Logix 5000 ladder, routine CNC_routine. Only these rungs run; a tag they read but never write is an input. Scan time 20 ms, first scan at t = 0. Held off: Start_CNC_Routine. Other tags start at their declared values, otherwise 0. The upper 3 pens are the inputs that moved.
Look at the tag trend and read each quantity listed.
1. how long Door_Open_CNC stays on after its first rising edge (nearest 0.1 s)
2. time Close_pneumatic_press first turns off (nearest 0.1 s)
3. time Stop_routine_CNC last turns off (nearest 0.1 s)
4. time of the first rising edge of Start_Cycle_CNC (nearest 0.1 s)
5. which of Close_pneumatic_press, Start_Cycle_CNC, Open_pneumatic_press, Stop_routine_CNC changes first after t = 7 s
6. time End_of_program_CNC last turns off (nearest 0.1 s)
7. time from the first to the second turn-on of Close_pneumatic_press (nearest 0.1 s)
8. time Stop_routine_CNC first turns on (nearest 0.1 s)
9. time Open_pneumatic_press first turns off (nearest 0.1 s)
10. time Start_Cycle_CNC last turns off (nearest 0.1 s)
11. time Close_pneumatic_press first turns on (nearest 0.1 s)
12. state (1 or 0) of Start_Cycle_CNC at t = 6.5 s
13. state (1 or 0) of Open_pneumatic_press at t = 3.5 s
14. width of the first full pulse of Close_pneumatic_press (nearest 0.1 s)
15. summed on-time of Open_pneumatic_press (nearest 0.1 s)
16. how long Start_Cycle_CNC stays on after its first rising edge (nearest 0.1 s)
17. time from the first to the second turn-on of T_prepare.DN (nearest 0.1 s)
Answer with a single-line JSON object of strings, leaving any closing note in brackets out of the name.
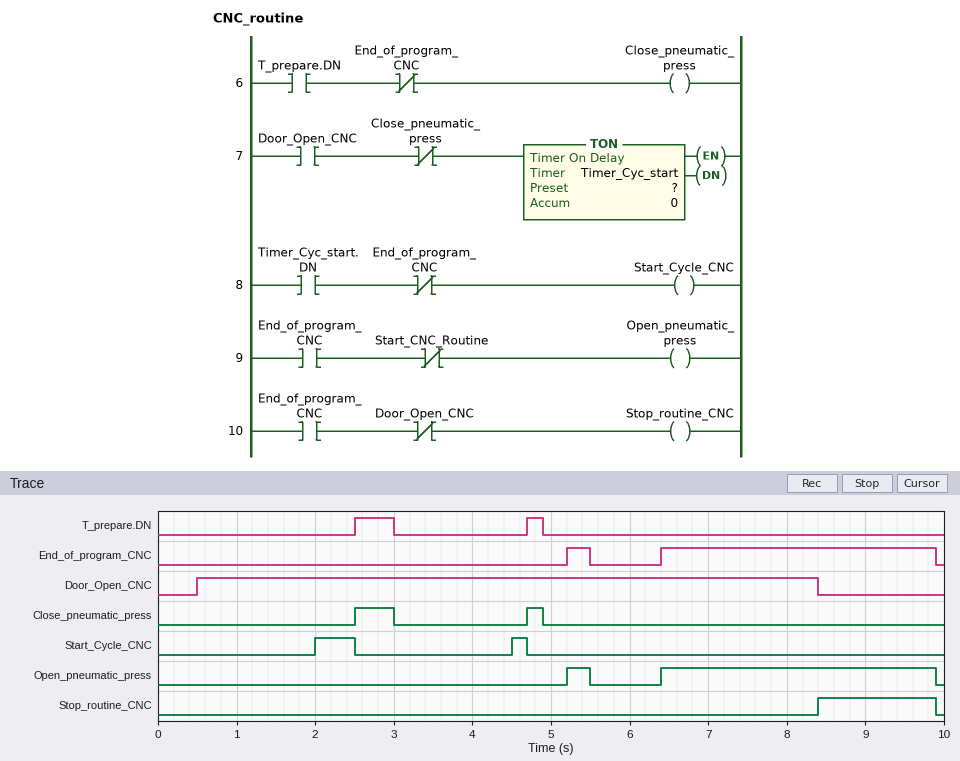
{"how long Door_Open_CNC stays on after its first rising edge": "7.9 s", "time Close_pneumatic_press first turns off": "3.0 s", "time Stop_routine_CNC last turns off": "9.9 s", "time of the first rising edge of Start_Cycle_CNC": "2.0 s", "which of Close_pneumatic_press, Start_Cycle_CNC, Open_pneumatic_press, Stop_routine_CNC changes first after t = 7 s": "Stop_routine_CNC", "time End_of_program_CNC last turns off": "9.9 s", "time from the first to the second turn-on of Close_pneumatic_press": "2.2 s", "time Stop_routine_CNC first turns on": "8.4 s", "time Open_pneumatic_press first turns off": "5.5 s", "time Start_Cycle_CNC last turns off": "4.7 s", "time Close_pneumatic_press first turns on": "2.5 s", "state (1 or 0) of Start_Cycle_CNC at t = 6.5 s": "0", "state (1 or 0) of Open_pneumatic_press at t = 3.5 s": "0", "width of the first full pulse of Close_pneumatic_press": "0.5 s", "summed on-time of Open_pneumatic_press": "3.8 s", "how long Start_Cycle_CNC stays on after its first rising edge": "0.5 s", "time from the first to the second turn-on of T_prepare.DN": "2.2 s"}
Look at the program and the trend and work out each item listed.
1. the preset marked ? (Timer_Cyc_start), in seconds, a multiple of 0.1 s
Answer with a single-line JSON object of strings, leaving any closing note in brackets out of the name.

{"the preset marked ? (Timer_Cyc_start), in seconds, a multiple of 0.1 s": "1.5 s"}
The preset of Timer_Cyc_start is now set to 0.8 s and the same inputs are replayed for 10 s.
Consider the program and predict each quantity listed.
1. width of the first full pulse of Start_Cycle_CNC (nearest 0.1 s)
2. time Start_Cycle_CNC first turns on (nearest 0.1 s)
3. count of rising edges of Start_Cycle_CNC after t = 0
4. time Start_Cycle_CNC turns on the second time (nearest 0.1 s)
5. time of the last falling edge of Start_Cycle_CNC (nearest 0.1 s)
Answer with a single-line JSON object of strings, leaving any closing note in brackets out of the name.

{"width of the first full pulse of Start_Cycle_CNC": "1.2 s", "time Start_Cycle_CNC first turns on": "1.3 s", "count of rising edges of Start_Cycle_CNC after t = 0": "3", "time Start_Cycle_CNC turns on the second time": "3.8 s", "time of the last falling edge of Start_Cycle_CNC": "6.4 s"}
